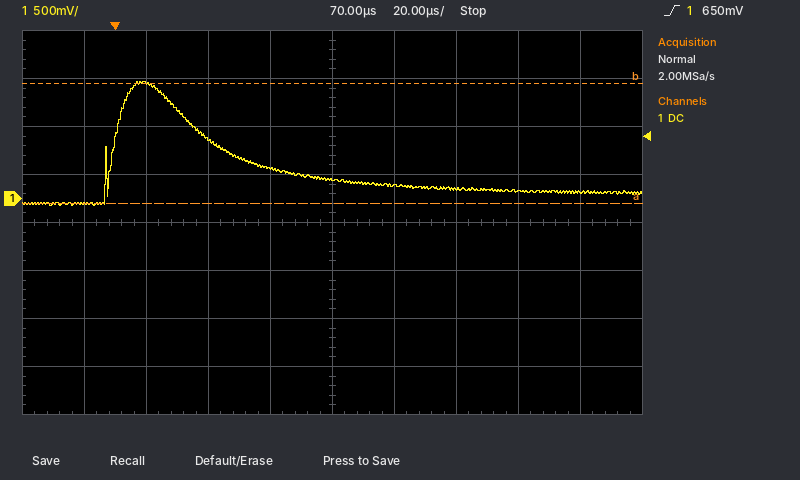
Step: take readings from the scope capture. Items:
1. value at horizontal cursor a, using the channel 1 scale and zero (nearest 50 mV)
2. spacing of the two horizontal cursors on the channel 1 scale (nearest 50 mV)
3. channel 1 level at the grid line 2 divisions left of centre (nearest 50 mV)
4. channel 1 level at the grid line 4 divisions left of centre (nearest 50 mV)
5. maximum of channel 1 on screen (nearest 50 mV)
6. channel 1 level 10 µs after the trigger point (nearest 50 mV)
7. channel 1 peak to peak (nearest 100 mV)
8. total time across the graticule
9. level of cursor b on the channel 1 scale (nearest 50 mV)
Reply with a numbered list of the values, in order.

1. -50 mV
2. 1.25 V
3. 600 mV
4. -50 mV
5. 1.20 V
6. 1.20 V
7. 1.30 V
8. 200 µs
9. 1.20 V
